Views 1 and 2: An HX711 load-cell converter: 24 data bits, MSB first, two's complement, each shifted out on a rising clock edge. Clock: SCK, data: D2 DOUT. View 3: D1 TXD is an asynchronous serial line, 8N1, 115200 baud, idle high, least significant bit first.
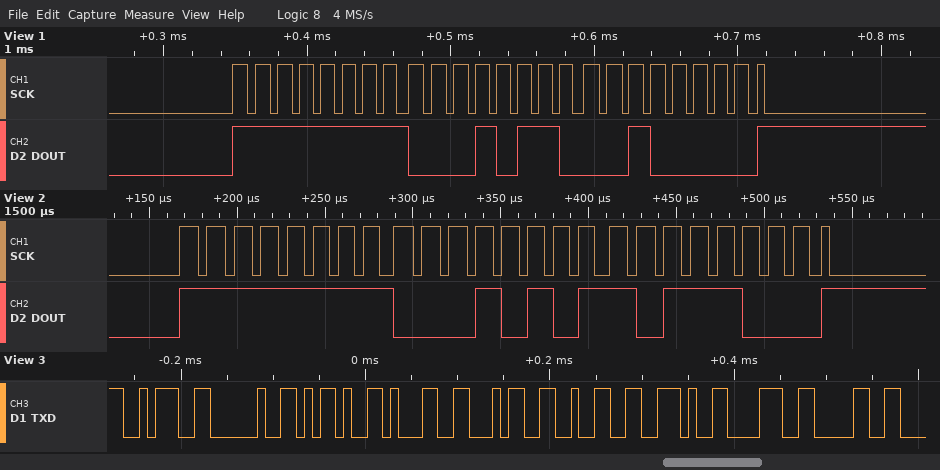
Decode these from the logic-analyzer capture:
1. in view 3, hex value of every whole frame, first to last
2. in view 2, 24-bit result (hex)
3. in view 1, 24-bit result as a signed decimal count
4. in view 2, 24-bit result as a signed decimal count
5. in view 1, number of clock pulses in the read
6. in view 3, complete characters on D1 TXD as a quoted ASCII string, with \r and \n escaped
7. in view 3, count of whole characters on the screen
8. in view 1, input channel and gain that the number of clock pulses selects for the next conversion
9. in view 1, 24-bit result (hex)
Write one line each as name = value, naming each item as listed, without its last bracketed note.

in view 3, hex value of every whole frame, first to last = 3A 20 2D 31 34 32 2E 38 30
in view 2, 24-bit result = 0xFF15B8
in view 1, 24-bit result as a signed decimal count = -59872
in view 2, 24-bit result as a signed decimal count = -59976
in view 1, number of clock pulses in the read = 25
in view 3, complete characters on D1 TXD as a quoted ASCII string, with \r and \n escaped = ": -142.80"
in view 3, count of whole characters on the screen = 9
in view 1, input channel and gain that the number of clock pulses selects for the next conversion = channel A, gain 128
in view 1, 24-bit result = 0xFF1620
